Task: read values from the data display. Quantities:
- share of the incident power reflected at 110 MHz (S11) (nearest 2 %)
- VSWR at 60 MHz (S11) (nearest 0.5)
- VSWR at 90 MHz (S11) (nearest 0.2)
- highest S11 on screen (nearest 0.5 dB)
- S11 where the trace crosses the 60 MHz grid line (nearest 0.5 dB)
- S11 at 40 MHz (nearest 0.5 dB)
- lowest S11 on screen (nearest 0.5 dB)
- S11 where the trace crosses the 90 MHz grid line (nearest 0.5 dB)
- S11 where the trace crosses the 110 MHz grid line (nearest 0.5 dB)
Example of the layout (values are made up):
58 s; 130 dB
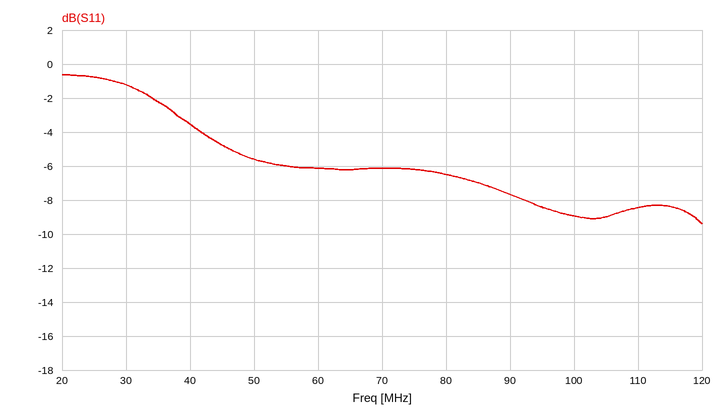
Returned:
14 %; 3.0; 2.4; -0.5 dB; -6.0 dB; -3.5 dB; -9.5 dB; -7.5 dB; -8.5 dB
